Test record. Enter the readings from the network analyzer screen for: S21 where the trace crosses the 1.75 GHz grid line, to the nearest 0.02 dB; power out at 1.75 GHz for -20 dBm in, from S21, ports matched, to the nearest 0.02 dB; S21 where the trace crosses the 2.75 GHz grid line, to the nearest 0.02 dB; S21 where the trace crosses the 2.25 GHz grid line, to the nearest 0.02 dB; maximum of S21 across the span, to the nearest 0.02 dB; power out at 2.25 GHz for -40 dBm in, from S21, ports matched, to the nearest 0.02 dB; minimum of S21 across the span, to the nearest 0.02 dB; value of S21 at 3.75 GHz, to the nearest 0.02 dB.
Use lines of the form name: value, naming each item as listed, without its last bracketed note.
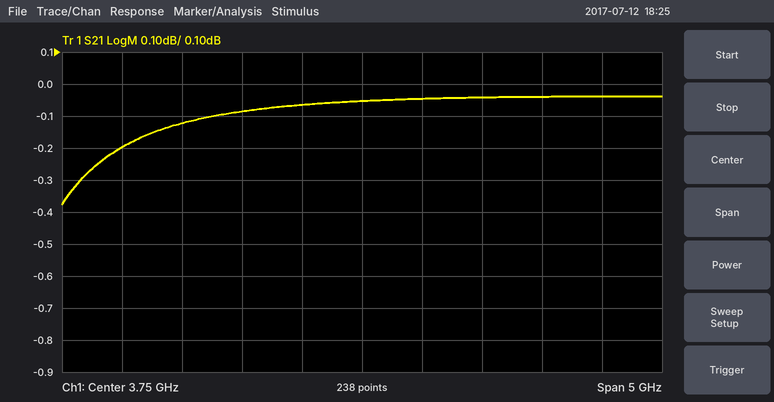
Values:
S21 where the trace crosses the 1.75 GHz grid line, to the nearest 0.02 dB: -0.20 dB
power out at 1.75 GHz for -20 dBm in, from S21, ports matched, to the nearest 0.02 dB: -20.20 dBm
S21 where the trace crosses the 2.75 GHz grid line, to the nearest 0.02 dB: -0.08 dB
S21 where the trace crosses the 2.25 GHz grid line, to the nearest 0.02 dB: -0.12 dB
maximum of S21 across the span, to the nearest 0.02 dB: -0.04 dB
power out at 2.25 GHz for -40 dBm in, from S21, ports matched, to the nearest 0.02 dB: -40.12 dBm
minimum of S21 across the span, to the nearest 0.02 dB: -0.38 dB
value of S21 at 3.75 GHz, to the nearest 0.02 dB: -0.06 dB
